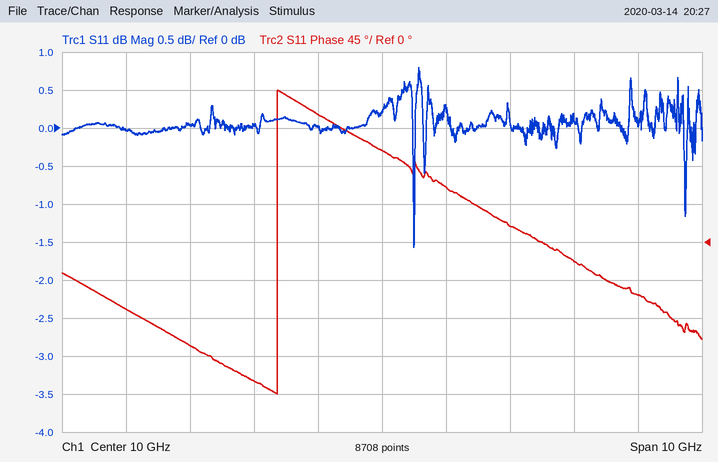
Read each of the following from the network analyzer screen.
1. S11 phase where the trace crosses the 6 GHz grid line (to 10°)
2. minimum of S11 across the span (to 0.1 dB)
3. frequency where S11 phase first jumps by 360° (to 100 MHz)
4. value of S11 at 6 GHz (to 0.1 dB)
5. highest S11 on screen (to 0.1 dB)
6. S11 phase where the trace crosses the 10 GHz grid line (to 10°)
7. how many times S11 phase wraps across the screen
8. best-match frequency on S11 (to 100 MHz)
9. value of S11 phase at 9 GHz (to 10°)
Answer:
-80°
-1.6 dB
8.4 GHz
0.0 dB
0.8 dB
110°
1
10.5 GHz
150°
